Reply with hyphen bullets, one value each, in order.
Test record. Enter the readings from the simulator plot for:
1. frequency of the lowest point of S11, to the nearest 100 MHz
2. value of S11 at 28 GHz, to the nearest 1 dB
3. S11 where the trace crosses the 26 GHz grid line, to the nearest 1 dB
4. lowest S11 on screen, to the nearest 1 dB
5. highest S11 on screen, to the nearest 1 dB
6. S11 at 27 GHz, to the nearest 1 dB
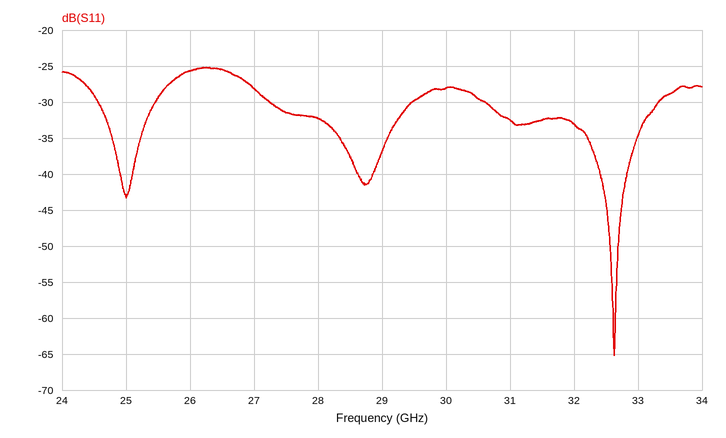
- 32.6 GHz
- -32 dB
- -26 dB
- -65 dB
- -25 dB
- -28 dB
